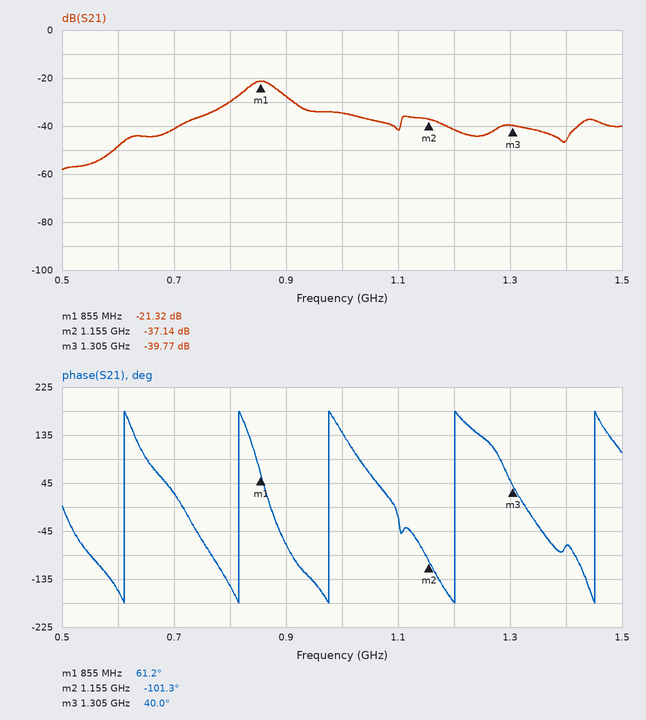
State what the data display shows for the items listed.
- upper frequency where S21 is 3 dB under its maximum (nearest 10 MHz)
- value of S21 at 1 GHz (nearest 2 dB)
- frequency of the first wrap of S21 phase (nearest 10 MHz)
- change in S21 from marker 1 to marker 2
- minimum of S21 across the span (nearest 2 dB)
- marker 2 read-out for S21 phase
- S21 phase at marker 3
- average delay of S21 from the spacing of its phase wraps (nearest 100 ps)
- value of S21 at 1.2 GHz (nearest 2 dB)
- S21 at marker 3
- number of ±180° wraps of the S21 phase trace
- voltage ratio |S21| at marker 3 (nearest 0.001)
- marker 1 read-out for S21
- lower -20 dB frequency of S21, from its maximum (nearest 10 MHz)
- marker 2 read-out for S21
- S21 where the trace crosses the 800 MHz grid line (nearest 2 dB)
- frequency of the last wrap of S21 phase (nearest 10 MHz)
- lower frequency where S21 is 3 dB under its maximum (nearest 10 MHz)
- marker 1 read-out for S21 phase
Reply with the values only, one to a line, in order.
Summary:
880 MHz
-34 dB
610 MHz
-15.82 dB
-58 dB
-101.3°
40.0°
4.8 ns
-42 dB
-39.77 dB
5
0.010
-21.32 dB
700 MHz
-37.14 dB
-30 dB
1.45 GHz
830 MHz
61.2°
